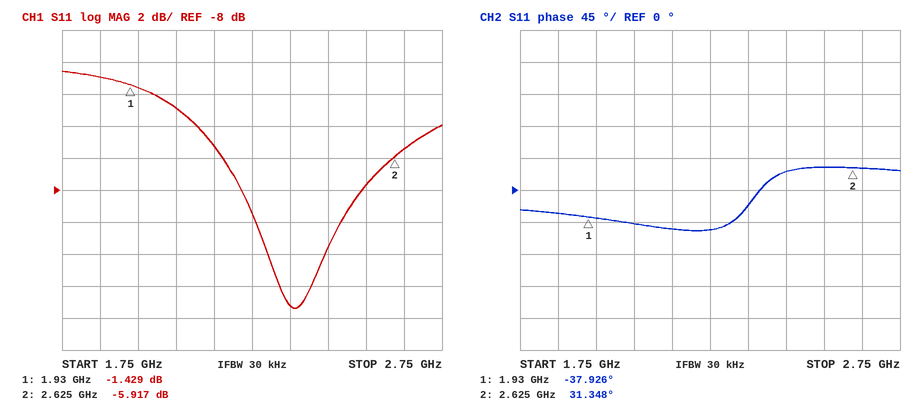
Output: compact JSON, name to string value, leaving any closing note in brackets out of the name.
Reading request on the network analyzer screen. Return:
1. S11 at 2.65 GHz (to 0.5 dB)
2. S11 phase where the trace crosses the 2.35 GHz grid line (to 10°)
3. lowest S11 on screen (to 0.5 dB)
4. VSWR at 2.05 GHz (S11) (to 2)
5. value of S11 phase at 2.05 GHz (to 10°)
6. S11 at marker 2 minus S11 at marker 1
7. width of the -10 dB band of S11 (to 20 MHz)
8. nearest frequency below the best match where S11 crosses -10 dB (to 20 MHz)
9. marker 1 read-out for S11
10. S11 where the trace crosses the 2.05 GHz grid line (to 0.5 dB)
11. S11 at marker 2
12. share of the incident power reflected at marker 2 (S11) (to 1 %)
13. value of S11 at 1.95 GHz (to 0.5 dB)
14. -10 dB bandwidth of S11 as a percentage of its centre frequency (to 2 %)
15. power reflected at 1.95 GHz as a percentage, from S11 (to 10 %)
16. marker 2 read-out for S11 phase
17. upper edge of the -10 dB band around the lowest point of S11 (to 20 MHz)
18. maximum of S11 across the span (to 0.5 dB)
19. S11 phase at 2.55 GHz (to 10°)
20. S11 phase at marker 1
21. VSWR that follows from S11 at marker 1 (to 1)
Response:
{"S11 at 2.65 GHz": "-5.5 dB", "S11 phase where the trace crosses the 2.35 GHz grid line": "-20°", "lowest S11 on screen": "-15.5 dB", "VSWR at 2.05 GHz (S11)": "6", "value of S11 phase at 2.05 GHz": "-50°", "S11 at marker 2 minus S11 at marker 1": "-4.488 dB", "width of the -10 dB band of S11": "220 MHz", "nearest frequency below the best match where S11 crosses -10 dB": "2.26 GHz", "marker 1 read-out for S11": "-1.429 dB", "S11 where the trace crosses the 2.05 GHz grid line": "-3.0 dB", "S11 at marker 2": "-5.917 dB", "share of the incident power reflected at marker 2 (S11)": "26 %", "value of S11 at 1.95 GHz": "-1.5 dB", "-10 dB bandwidth of S11 as a percentage of its centre frequency": "10 %", "power reflected at 1.95 GHz as a percentage, from S11": "70 %", "marker 2 read-out for S11 phase": "31.348°", "upper edge of the -10 dB band around the lowest point of S11": "2.48 GHz", "maximum of S11 across the span": "-0.5 dB", "S11 phase at 2.55 GHz": "30°", "S11 phase at marker 1": "-37.926°", "VSWR that follows from S11 at marker 1": "12"}
